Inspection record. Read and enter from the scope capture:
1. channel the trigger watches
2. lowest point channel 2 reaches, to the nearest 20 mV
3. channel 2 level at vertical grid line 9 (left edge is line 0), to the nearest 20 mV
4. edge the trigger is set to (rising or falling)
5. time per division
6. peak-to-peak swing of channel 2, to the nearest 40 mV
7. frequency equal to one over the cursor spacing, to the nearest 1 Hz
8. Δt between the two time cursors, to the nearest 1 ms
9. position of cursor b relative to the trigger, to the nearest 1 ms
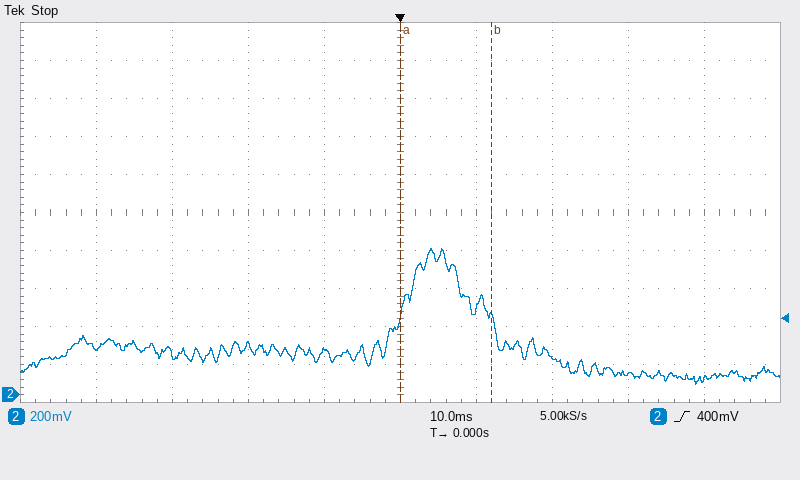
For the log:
channel 2
60 mV
80 mV
rising
10 ms
720 mV
83 Hz
12 ms
+12 ms
